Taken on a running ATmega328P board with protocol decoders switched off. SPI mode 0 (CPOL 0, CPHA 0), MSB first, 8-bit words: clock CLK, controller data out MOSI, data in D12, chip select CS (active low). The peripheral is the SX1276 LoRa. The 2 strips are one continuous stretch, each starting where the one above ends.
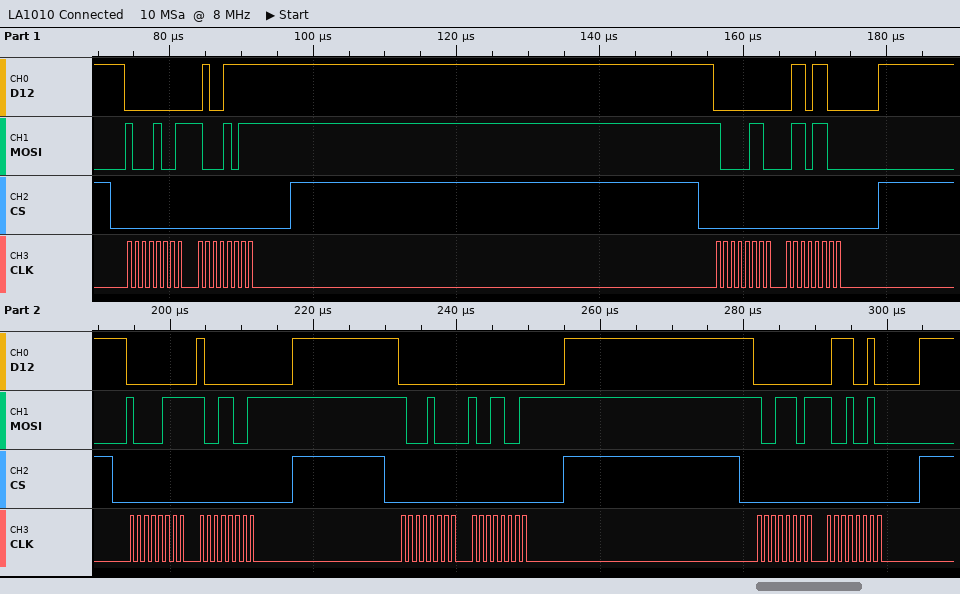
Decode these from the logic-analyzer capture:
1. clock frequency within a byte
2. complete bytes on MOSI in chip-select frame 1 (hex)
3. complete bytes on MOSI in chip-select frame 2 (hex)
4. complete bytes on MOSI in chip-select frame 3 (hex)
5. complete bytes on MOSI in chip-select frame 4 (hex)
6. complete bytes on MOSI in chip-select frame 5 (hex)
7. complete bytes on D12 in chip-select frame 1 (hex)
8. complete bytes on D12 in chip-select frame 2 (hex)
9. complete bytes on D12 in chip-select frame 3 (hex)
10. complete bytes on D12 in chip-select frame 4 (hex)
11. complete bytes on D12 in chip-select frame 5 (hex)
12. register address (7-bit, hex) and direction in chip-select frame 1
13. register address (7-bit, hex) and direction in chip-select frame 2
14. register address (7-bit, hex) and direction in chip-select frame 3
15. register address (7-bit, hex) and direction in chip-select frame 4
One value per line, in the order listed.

1 MHz
89 8B
86 6C
87 99
88 99
9D 92
00 4F
00 6C
00 80
00 00
00 72
0x09 write
0x06 write
0x07 write
0x08 write
